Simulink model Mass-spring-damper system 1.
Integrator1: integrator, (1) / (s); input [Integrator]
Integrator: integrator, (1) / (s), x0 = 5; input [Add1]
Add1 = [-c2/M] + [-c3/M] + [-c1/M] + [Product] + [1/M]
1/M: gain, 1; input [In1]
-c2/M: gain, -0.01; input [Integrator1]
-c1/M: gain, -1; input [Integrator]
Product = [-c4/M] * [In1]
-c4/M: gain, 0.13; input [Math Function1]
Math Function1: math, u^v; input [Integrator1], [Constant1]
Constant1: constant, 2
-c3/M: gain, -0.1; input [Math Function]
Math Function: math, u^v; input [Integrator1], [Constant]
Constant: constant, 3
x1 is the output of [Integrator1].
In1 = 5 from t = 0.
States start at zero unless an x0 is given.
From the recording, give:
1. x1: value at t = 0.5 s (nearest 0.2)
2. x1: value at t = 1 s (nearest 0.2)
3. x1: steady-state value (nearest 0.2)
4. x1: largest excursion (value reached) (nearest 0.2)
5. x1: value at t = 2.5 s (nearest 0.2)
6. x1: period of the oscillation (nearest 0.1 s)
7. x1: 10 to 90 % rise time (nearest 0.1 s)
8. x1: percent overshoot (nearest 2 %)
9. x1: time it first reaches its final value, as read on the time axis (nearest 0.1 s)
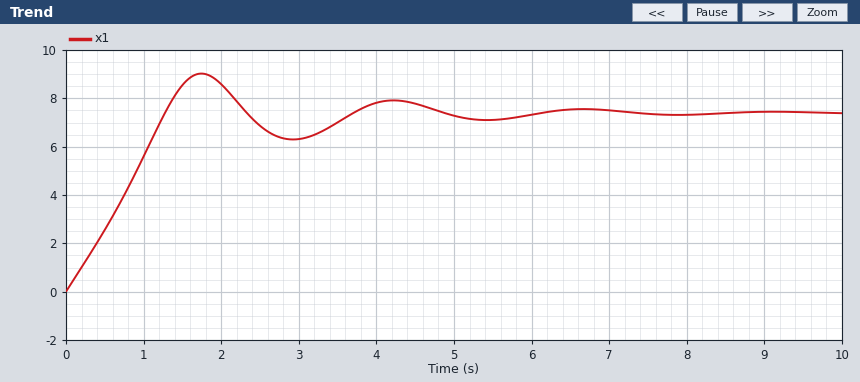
2.6
5.6
7.4
9.0
6.8
2.5 s
1.0 s
22 %
1.3 s
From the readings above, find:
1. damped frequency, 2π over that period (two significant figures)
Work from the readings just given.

2.5 rad/s
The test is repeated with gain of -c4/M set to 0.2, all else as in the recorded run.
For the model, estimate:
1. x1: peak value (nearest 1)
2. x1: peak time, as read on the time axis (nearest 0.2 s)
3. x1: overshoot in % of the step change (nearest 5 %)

13
1.8 s
20 %
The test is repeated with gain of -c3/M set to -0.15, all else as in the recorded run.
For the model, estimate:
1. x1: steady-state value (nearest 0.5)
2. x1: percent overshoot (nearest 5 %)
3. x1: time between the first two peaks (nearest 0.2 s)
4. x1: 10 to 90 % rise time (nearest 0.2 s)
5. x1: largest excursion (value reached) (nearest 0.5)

5.5
25 %
2.6 s
0.8 s
7.0
